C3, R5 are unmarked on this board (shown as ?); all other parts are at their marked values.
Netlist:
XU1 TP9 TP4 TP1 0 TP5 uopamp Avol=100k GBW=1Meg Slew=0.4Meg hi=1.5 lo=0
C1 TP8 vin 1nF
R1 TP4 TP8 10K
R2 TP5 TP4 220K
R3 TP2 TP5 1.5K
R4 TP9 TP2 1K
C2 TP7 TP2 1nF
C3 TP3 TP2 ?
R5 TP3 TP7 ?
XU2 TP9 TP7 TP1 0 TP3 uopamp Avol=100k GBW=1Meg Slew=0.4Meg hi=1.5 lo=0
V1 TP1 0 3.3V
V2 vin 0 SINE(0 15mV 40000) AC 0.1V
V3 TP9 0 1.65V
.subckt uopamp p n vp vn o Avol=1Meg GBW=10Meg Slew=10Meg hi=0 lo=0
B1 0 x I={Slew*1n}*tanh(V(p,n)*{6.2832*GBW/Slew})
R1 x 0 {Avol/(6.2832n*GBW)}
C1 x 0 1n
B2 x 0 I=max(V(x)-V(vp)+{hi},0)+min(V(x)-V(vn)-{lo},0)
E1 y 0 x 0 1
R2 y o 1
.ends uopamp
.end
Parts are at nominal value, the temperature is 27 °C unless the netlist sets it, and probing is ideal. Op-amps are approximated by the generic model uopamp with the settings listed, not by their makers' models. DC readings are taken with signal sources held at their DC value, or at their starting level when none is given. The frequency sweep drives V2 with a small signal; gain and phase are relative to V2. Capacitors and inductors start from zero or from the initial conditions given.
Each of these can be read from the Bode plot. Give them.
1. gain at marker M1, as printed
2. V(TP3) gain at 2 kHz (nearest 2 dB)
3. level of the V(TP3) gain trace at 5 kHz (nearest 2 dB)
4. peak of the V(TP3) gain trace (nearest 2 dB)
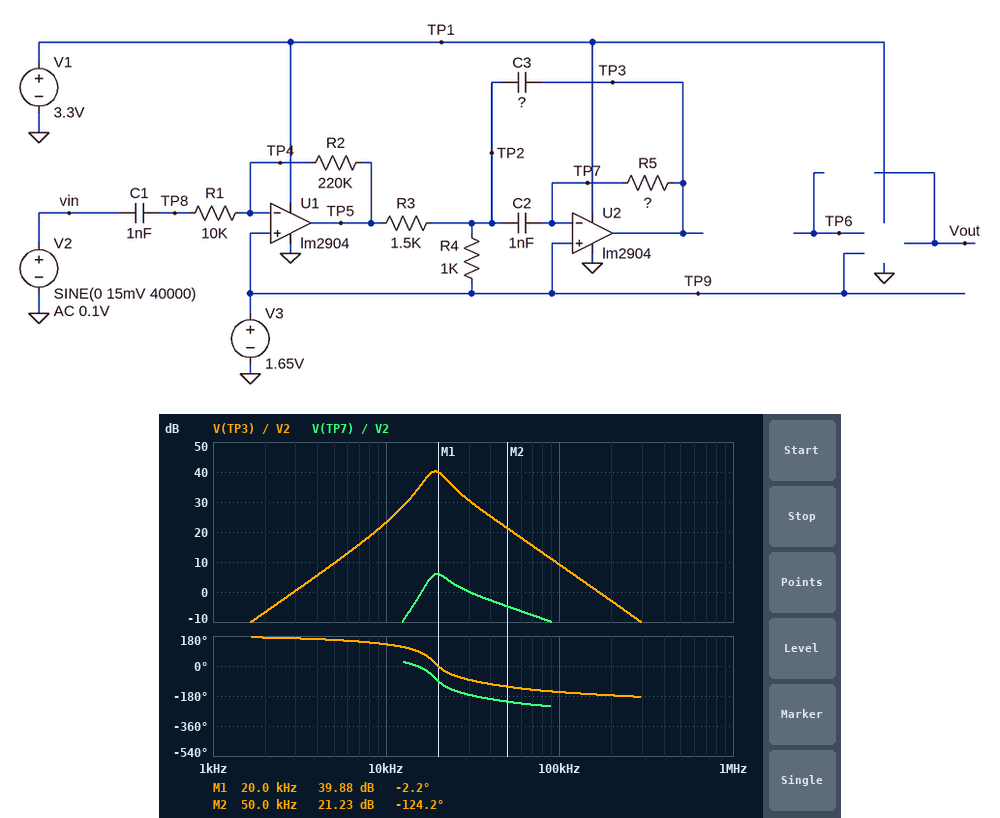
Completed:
39.88 dB
-6 dB
10 dB
40 dB
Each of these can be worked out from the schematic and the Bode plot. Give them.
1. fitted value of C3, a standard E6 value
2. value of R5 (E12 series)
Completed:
3.3 nF
33 kΩ
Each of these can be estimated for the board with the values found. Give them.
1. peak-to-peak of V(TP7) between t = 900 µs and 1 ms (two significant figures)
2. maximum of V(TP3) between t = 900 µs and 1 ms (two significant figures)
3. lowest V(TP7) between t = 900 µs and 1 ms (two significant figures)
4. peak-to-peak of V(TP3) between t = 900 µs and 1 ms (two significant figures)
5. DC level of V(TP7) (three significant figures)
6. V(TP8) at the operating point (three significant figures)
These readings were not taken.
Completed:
46 mV
1.8 V
1.6 V
330 mV
1.65 V
1.65 V
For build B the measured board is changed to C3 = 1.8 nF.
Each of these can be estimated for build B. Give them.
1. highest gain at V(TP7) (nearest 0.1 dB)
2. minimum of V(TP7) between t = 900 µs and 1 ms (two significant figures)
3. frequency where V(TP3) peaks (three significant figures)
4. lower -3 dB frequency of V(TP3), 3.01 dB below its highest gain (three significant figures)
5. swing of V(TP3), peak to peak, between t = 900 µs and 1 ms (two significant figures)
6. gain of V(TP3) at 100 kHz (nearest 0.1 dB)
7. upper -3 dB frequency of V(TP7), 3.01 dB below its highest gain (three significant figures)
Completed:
12.5 dB
1.5 V
24.9 kHz
21.9 kHz
420 mV
14.1 dB
29.6 kHz
